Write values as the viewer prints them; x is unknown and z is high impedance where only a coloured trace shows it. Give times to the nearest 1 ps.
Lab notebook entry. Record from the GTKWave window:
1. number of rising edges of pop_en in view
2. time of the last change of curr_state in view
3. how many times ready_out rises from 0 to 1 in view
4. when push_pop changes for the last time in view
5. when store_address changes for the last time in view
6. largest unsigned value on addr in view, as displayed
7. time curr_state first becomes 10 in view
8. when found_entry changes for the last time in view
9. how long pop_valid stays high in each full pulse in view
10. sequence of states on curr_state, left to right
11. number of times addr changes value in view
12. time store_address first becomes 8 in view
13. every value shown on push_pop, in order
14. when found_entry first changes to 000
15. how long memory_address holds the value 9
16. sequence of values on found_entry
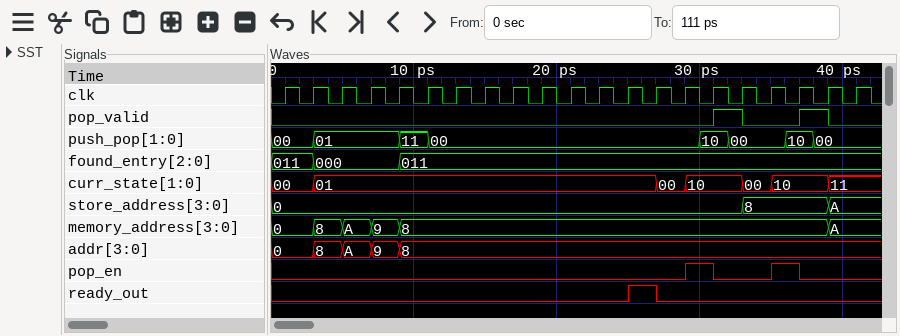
2
39 ps
1
38 ps
39 ps
A
29 ps
9 ps
2 ps, 2 ps
00, 01, 00, 10, 00, 10, 11
4
33 ps
00, 01, 11, 00, 10, 00, 10, 00
3 ps
2 ps
011, 000, 011
